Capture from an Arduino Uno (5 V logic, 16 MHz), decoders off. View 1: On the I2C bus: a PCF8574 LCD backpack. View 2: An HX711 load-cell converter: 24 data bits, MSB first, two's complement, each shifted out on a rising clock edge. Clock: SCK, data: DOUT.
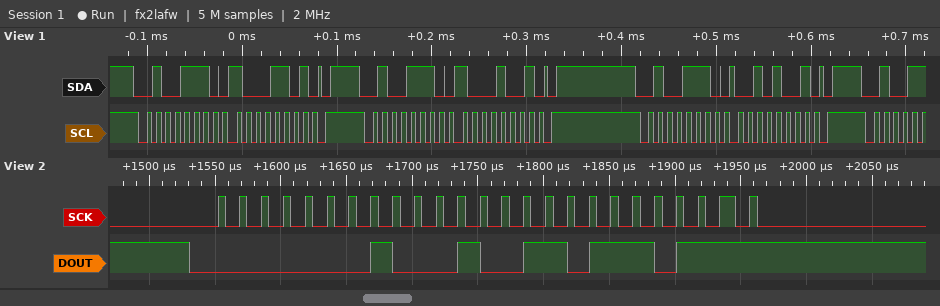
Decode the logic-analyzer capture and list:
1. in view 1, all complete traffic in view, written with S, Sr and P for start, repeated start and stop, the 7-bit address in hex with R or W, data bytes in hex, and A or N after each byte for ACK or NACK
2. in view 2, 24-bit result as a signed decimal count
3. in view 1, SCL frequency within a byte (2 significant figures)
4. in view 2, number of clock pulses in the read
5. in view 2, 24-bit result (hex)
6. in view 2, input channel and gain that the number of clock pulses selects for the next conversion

S 27W A 8D A P S 27W A 89 A P S 27W A 29 A P
70519
100 kHz
25
0x011377
channel A, gain 128
